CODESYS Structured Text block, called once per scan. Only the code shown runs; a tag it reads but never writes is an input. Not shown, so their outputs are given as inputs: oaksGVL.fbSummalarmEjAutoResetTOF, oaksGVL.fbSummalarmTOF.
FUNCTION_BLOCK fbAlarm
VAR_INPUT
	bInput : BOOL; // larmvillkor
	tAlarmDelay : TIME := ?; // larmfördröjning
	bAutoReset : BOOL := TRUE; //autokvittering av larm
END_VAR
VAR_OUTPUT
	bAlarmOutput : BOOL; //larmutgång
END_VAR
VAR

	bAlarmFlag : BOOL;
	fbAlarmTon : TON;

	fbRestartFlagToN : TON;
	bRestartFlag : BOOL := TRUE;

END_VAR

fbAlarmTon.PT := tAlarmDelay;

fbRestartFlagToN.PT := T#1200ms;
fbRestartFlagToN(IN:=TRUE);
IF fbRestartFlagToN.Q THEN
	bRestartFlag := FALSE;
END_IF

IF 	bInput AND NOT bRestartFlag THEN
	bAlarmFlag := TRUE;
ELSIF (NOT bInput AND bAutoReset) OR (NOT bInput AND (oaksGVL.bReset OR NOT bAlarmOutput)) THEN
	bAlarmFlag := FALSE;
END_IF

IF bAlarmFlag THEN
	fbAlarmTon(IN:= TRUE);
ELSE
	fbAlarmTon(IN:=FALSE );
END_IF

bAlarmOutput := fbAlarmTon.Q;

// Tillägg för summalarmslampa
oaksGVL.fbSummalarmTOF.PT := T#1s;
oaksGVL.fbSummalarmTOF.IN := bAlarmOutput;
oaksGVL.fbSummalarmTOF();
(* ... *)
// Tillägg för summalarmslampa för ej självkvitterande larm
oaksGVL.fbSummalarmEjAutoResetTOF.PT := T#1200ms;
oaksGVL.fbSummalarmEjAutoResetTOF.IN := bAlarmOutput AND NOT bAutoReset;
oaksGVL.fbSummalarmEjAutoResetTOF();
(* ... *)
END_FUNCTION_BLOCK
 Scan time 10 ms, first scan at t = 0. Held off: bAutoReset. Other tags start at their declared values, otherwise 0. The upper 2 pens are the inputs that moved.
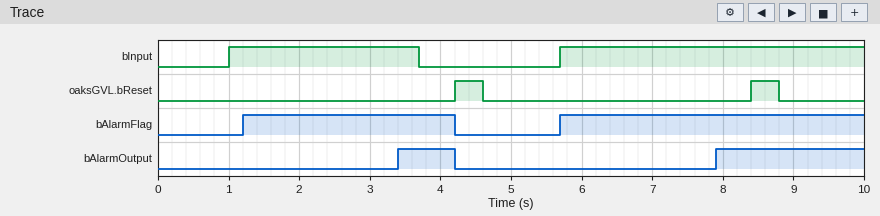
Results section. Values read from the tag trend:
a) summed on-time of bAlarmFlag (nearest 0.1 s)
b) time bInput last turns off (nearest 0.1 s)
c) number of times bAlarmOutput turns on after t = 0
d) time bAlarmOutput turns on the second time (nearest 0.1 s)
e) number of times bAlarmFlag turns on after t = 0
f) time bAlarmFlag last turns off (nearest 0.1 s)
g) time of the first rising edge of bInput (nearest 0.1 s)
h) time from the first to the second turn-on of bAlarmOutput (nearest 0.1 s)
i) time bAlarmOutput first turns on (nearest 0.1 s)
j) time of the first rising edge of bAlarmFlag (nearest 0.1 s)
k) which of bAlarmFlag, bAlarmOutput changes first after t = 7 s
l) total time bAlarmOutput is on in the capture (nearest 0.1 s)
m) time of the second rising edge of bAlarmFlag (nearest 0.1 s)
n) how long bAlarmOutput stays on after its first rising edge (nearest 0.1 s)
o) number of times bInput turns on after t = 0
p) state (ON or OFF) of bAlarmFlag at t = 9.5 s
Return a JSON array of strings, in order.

["7.3 s", "3.7 s", "2", "7.9 s", "2", "4.2 s", "1.0 s", "4.5 s", "3.4 s", "1.2 s", "bAlarmOutput", "2.9 s", "5.7 s", "0.8 s", "2", "ON"]
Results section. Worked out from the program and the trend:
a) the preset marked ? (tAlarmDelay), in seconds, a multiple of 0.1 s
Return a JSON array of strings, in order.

["2.2 s"]
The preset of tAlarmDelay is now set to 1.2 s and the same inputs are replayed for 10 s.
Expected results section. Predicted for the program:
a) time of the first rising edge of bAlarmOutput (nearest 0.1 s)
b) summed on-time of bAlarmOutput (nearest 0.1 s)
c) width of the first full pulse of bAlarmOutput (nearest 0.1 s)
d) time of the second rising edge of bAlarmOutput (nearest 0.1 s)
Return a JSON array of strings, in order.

["2.4 s", "4.9 s", "1.8 s", "6.9 s"]
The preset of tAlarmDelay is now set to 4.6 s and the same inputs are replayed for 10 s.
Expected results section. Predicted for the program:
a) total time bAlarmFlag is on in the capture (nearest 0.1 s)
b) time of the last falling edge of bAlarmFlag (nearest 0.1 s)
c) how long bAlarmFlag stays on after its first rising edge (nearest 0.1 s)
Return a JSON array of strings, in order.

["6.8 s", "3.7 s", "2.5 s"]
